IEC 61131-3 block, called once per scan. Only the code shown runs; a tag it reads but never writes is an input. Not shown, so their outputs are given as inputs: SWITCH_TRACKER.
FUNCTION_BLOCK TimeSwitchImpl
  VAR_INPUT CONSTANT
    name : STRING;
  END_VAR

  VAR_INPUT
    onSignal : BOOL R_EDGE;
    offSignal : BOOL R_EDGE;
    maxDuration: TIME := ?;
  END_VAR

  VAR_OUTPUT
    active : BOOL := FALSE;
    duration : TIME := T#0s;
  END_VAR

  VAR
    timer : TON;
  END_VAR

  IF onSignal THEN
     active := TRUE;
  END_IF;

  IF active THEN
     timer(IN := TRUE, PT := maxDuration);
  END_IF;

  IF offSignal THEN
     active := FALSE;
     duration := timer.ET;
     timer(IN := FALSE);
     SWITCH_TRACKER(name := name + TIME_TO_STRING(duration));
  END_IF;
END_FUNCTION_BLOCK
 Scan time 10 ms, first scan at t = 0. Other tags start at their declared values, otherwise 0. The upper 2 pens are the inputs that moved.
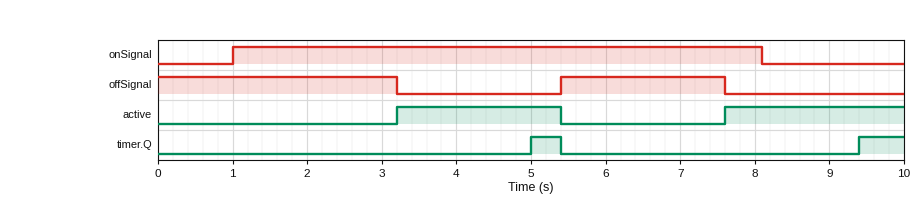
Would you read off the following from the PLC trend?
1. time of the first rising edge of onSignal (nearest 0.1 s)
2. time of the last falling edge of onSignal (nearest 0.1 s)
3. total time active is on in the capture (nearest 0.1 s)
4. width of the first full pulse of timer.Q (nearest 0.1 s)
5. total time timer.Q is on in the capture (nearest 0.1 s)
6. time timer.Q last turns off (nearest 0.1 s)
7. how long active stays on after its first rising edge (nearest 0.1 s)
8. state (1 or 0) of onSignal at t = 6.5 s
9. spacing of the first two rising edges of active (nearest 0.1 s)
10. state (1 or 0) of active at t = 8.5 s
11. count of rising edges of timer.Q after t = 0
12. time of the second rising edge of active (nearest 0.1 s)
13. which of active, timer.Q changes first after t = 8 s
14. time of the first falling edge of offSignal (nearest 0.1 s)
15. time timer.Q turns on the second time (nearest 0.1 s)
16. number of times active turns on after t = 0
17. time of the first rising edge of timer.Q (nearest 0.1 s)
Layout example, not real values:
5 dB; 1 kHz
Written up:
1.0 s; 8.1 s; 4.6 s; 0.4 s; 1.0 s; 5.4 s; 2.2 s; 1; 4.4 s; 1; 2; 7.6 s; timer.Q; 3.2 s; 9.4 s; 2; 5.0 s
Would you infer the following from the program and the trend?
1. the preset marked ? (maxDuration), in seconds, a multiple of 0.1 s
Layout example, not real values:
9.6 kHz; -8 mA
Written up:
1.8 s
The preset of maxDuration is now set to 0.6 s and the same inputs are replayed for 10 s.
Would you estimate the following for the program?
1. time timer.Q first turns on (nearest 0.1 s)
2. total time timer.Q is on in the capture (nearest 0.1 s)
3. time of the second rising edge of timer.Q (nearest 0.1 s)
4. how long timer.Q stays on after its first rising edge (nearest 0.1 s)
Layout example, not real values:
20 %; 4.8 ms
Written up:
3.8 s; 3.4 s; 8.2 s; 1.6 s
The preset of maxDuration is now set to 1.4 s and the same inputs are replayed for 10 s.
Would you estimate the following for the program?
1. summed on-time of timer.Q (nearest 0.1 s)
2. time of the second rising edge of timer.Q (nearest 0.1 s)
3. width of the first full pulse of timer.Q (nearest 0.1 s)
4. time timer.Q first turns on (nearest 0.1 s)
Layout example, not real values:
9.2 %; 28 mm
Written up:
1.8 s; 9.0 s; 0.8 s; 4.6 s
